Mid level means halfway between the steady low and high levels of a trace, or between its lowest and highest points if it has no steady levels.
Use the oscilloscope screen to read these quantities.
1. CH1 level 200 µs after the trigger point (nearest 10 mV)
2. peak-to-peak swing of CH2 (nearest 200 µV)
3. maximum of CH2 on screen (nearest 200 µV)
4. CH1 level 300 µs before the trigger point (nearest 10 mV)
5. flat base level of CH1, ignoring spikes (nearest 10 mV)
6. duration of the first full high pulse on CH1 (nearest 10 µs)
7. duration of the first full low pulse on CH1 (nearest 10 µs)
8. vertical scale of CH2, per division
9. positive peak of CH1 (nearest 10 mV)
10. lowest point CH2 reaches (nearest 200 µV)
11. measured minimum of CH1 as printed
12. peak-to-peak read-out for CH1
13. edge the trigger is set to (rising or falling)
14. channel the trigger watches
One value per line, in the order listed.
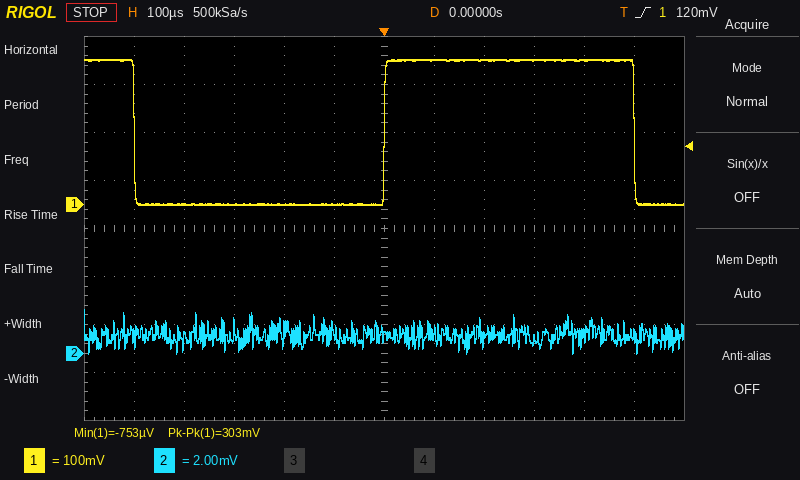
300 mV
1.8 mV
1.8 mV
0 mV
0 mV
500 µs
500 µs
2 mV
300 mV
0.0 mV
-753 µV
303 mV
rising
CH1
